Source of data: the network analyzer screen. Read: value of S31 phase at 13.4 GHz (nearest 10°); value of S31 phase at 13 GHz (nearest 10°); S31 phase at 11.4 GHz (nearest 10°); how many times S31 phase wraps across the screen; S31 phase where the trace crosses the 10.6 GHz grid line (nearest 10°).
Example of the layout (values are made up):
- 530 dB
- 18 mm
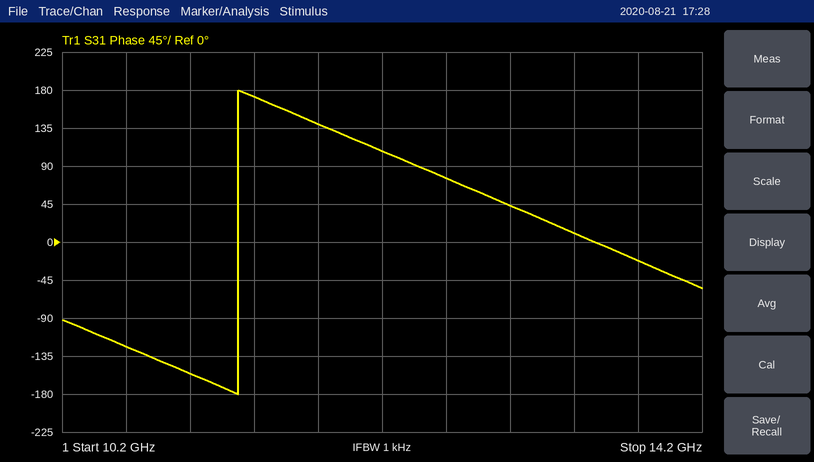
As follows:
- 10°
- 40°
- 170°
- 1
- -120°
